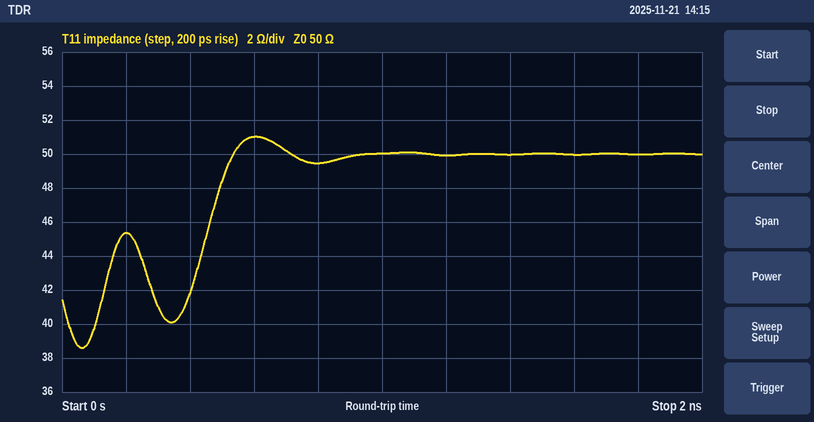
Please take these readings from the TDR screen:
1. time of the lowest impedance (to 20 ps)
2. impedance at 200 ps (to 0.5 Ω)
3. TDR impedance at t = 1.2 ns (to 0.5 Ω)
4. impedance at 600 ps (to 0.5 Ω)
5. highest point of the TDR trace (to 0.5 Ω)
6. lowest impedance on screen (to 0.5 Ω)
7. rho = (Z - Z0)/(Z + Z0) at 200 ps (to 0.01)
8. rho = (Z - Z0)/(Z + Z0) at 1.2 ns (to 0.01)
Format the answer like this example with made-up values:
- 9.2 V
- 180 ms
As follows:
- 60 ps
- 45.5 Ω
- 50.0 Ω
- 51.0 Ω
- 51.0 Ω
- 38.5 Ω
- -0.05
- 0.00
